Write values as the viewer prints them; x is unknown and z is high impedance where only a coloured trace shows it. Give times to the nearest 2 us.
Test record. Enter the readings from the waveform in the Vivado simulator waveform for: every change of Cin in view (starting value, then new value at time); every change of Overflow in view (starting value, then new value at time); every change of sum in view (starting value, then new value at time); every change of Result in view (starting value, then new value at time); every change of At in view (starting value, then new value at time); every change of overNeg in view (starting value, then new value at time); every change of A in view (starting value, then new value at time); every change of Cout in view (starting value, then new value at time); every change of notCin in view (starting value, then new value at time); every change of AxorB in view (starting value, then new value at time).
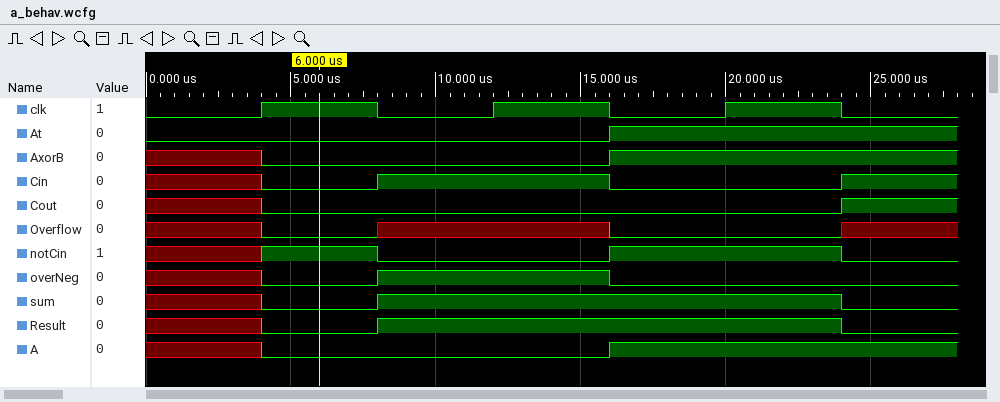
x, 0 at 4 us, 1 at 8 us, 0 at 16 us, 1 at 24 us
x, 0 at 4 us, x at 8 us, 0 at 16 us, x at 24 us
x, 0 at 4 us, 1 at 8 us, 0 at 24 us
x, 0 at 4 us, 1 at 8 us, 0 at 24 us
0, 1 at 16 us
x, 0 at 4 us, 1 at 8 us, 0 at 16 us
x, 0 at 4 us, 1 at 16 us
x, 0 at 4 us, 1 at 24 us
x, 1 at 4 us, 0 at 8 us, 1 at 16 us, 0 at 24 us
x, 0 at 4 us, 1 at 16 us
